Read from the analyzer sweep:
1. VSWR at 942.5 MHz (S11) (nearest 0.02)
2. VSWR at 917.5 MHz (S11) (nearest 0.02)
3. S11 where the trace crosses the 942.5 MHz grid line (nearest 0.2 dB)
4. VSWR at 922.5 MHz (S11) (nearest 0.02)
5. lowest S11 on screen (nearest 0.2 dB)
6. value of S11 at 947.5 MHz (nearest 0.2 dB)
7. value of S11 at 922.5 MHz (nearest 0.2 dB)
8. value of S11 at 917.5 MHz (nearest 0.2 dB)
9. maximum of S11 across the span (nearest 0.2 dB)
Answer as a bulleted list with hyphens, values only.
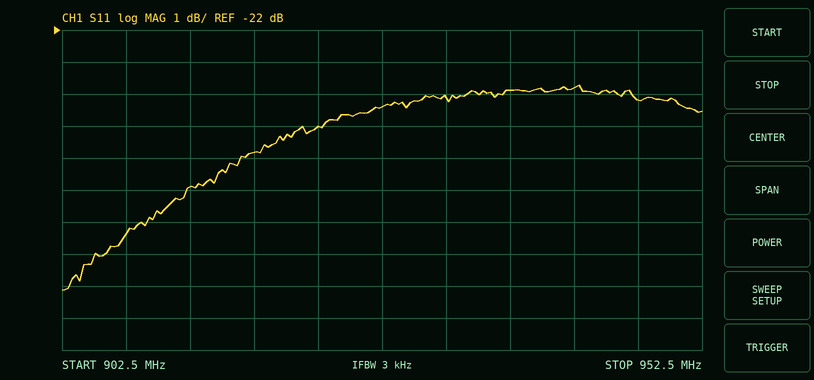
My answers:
- 1.14
- 1.10
- -23.8 dB
- 1.12
- -30.2 dB
- -24.2 dB
- -25.0 dB
- -25.8 dB
- -23.8 dB
